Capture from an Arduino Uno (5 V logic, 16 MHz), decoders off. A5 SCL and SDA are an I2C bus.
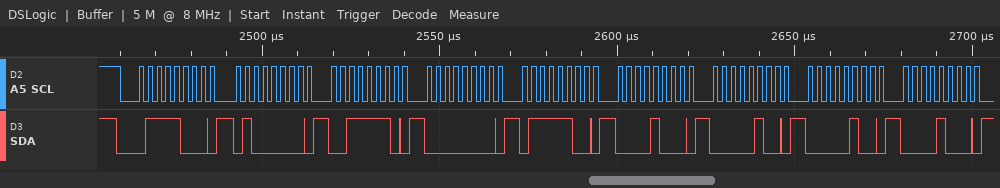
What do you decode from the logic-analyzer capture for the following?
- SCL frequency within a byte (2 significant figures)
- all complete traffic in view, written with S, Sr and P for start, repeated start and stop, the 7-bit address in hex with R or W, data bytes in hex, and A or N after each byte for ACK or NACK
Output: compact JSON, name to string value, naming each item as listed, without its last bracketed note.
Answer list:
{"SCL frequency within a byte": "400 kHz", "all complete traffic in view, written with S, Sr and P for start, repeated start and stop, the 7-bit address in hex with R or W, data bytes in hex, and A or N after each byte for ACK or NACK": "S 3CW A 40 A 3E A 00 A 7C A 08 A 04 A 04 A 08 A"}
